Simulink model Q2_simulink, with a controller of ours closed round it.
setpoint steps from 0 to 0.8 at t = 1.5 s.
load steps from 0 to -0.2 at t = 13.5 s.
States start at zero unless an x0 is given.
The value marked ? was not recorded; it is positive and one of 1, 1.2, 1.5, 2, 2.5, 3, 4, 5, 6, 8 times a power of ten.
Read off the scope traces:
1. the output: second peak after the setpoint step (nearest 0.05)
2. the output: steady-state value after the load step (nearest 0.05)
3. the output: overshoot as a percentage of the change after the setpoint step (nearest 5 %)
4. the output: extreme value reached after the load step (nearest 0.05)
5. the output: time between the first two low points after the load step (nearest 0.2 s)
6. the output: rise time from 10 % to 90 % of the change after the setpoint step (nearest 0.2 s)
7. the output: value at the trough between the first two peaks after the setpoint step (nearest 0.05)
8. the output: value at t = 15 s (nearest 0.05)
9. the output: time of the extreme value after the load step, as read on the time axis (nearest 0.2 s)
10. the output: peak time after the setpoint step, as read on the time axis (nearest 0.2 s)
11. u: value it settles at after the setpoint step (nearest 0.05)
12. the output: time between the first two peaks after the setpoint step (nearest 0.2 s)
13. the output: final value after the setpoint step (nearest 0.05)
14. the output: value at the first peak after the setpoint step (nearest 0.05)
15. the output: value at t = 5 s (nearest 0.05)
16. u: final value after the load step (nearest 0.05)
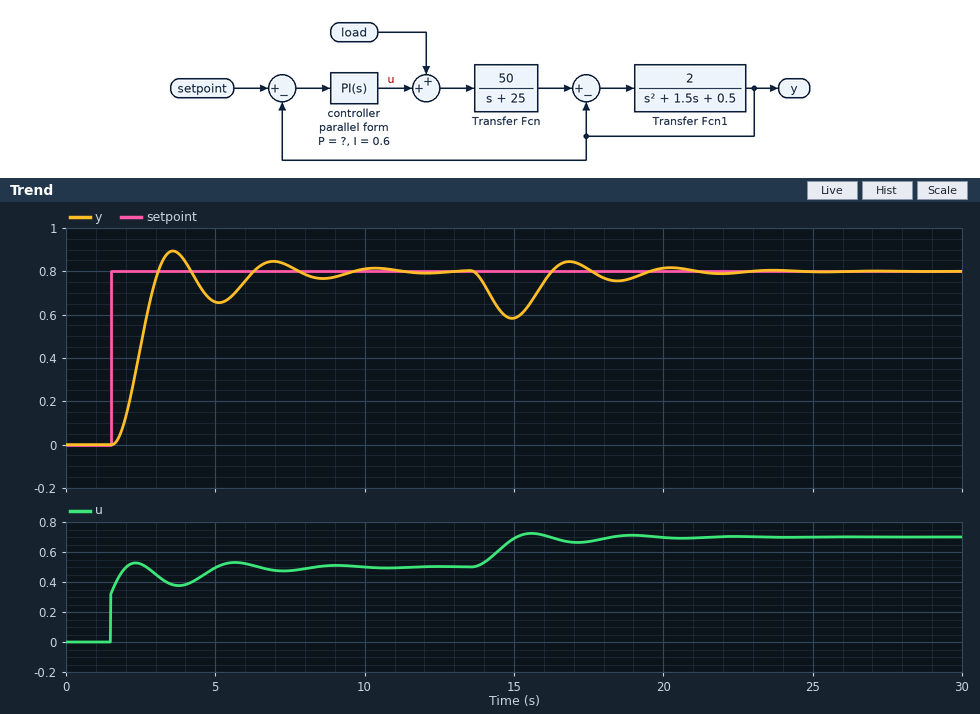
0.85
0.80
10 %
0.60
3.6 s
1.0 s
0.65
0.60
15.0 s
3.6 s
0.50
3.4 s
0.80
0.90
0.65
0.70
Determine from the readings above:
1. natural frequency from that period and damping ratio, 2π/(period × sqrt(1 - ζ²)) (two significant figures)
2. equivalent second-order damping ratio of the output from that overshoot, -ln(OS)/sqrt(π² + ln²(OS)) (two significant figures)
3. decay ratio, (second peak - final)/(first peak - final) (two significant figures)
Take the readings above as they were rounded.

2.3 rad/s
0.59
0.50
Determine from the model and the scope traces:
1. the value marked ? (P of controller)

0.4
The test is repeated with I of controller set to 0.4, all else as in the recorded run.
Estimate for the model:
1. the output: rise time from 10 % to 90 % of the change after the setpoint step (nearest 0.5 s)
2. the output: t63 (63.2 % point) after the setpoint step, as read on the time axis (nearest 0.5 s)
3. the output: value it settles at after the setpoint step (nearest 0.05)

1.5 s
2.5 s
0.80
